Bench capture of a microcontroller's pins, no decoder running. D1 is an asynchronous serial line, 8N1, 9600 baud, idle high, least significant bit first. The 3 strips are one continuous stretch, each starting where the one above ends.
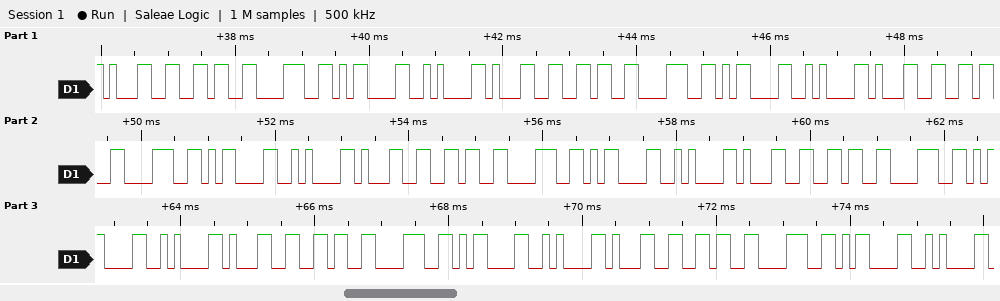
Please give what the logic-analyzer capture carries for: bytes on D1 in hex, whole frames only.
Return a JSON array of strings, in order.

["31 36 38 0D 0A 31 36 38 0D 0A 31 36 38 0D 0A 31 36 38 0D 0A 31 36 38 0D 0A 31 36 38 0D 0A 31 36 38 0D 0A"]
